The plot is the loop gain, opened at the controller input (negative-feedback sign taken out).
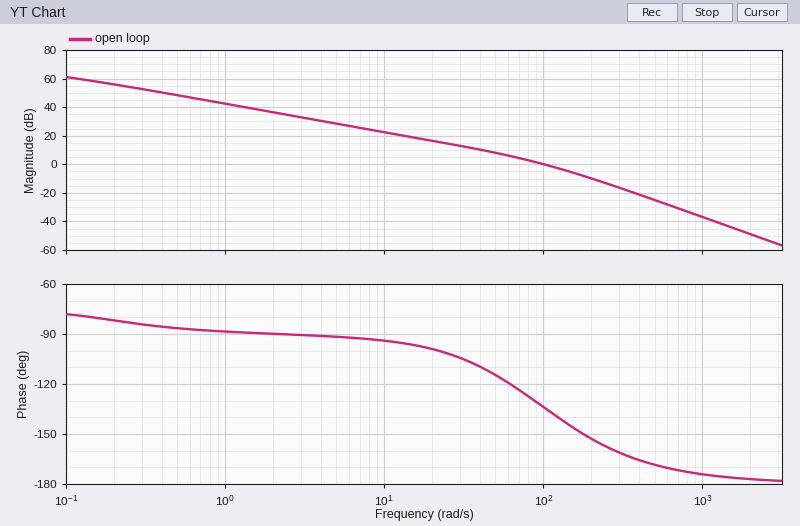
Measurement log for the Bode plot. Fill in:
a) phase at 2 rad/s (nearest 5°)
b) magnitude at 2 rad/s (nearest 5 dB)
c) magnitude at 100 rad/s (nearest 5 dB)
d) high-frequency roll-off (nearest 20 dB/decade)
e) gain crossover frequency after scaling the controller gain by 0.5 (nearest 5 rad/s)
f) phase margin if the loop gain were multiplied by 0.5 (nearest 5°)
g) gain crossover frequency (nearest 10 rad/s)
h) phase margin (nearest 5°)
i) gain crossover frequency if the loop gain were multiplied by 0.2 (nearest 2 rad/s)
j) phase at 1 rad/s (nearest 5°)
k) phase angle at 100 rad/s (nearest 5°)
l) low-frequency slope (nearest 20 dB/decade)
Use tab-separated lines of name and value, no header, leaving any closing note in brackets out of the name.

phase at 2 rad/s	-90°
magnitude at 2 rad/s	35 dB
magnitude at 100 rad/s	0 dB
high-frequency roll-off	-40 dB/decade
gain crossover frequency after scaling the controller gain by 0.5	60 rad/s
phase margin if the loop gain were multiplied by 0.5	60°
gain crossover frequency	100 rad/s
phase margin	45°
gain crossover frequency if the loop gain were multiplied by 0.2	26 rad/s
phase at 1 rad/s	-90°
phase angle at 100 rad/s	-135°
low-frequency slope	-20 dB/decade
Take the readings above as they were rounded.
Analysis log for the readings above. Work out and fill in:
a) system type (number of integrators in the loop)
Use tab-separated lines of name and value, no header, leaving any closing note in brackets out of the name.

system type	1
